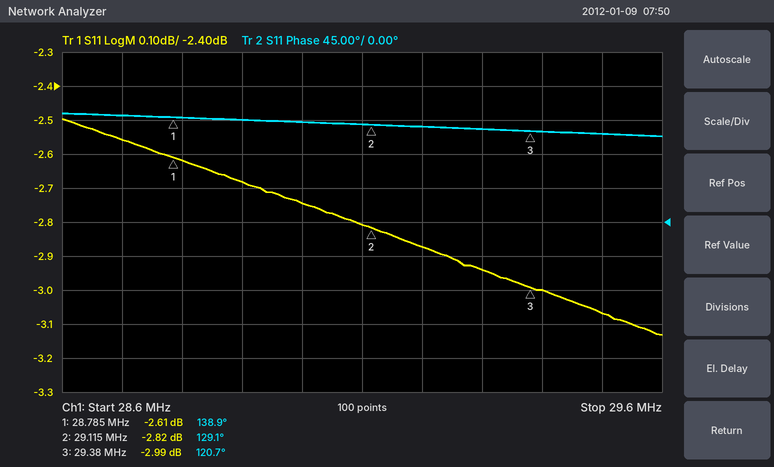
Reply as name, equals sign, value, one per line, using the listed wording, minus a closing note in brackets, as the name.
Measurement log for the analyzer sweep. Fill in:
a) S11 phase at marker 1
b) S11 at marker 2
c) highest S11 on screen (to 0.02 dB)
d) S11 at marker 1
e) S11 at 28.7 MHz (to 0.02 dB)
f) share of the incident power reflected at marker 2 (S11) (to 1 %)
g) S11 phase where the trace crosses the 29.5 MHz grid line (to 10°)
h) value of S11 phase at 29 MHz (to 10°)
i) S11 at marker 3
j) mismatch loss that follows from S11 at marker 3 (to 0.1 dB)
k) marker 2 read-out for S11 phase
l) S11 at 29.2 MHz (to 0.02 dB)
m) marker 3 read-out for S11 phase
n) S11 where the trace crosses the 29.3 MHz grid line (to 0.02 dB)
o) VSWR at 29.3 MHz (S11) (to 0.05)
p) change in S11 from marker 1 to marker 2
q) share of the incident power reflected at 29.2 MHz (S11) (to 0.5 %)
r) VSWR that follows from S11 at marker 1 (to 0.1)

S11 phase at marker 1 = 138.9°
S11 at marker 2 = -2.82 dB
highest S11 on screen = -2.50 dB
S11 at marker 1 = -2.61 dB
S11 at 28.7 MHz = -2.56 dB
share of the incident power reflected at marker 2 (S11) = 52 %
S11 phase where the trace crosses the 29.5 MHz grid line = 120°
value of S11 phase at 29 MHz = 130°
S11 at marker 3 = -2.99 dB
mismatch loss that follows from S11 at marker 3 = 3.0 dB
marker 2 read-out for S11 phase = 129.1°
S11 at 29.2 MHz = -2.88 dB
marker 3 read-out for S11 phase = 120.7°
S11 where the trace crosses the 29.3 MHz grid line = -2.94 dB
VSWR at 29.3 MHz (S11) = 5.95
change in S11 from marker 1 to marker 2 = -0.21 dB
share of the incident power reflected at 29.2 MHz (S11) = 51.5 %
VSWR that follows from S11 at marker 1 = 6.7
